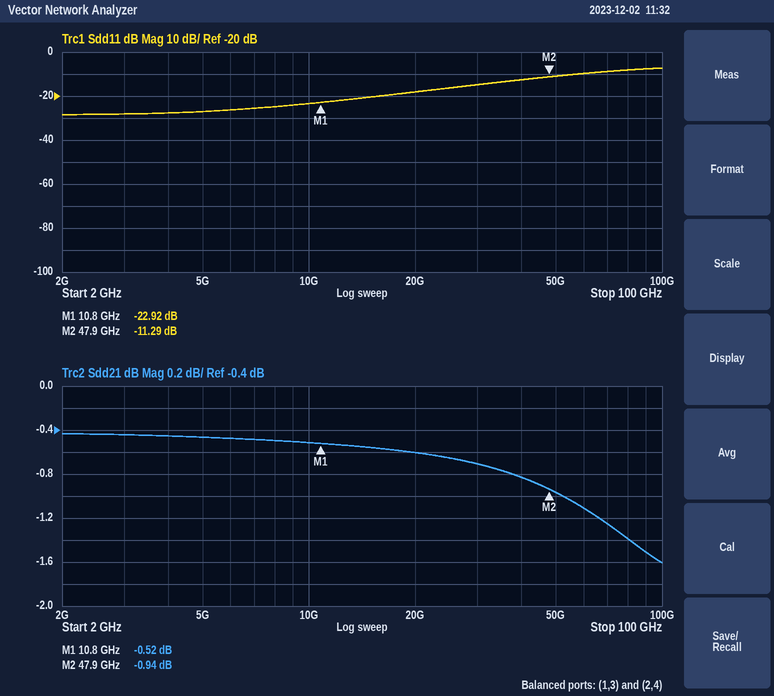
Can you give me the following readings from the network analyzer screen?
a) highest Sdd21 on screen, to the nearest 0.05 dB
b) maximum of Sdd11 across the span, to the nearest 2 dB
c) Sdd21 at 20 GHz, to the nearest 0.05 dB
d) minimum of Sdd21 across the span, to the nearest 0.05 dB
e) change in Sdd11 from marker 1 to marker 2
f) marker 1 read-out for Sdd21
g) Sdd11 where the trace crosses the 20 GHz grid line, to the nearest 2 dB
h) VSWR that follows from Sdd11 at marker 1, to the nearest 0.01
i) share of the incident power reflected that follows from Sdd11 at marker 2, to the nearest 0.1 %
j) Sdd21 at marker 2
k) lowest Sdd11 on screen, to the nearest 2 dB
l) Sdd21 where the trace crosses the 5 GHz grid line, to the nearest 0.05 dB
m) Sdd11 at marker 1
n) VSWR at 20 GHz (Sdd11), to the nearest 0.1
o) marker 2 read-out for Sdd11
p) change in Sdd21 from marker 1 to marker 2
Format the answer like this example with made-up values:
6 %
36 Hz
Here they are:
-0.45 dB
-8 dB
-0.60 dB
-1.60 dB
11.63 dB
-0.52 dB
-18 dB
1.15
7.4 %
-0.94 dB
-28 dB
-0.45 dB
-22.92 dB
1.3
-11.29 dB
-0.42 dB
